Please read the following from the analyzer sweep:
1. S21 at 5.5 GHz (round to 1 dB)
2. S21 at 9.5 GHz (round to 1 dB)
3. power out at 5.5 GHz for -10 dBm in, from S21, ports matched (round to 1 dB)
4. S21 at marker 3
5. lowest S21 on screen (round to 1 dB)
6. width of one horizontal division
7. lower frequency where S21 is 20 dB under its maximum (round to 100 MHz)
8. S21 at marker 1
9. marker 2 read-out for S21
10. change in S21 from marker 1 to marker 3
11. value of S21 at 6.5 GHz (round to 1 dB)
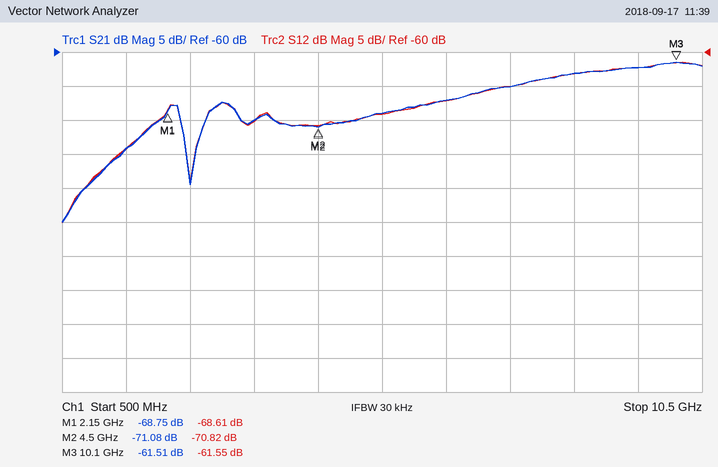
-69 dB
-62 dB
-79 dBm
-61.51 dB
-85 dB
1 GHz
700 MHz
-68.75 dB
-71.08 dB
7.24 dB
-67 dB
